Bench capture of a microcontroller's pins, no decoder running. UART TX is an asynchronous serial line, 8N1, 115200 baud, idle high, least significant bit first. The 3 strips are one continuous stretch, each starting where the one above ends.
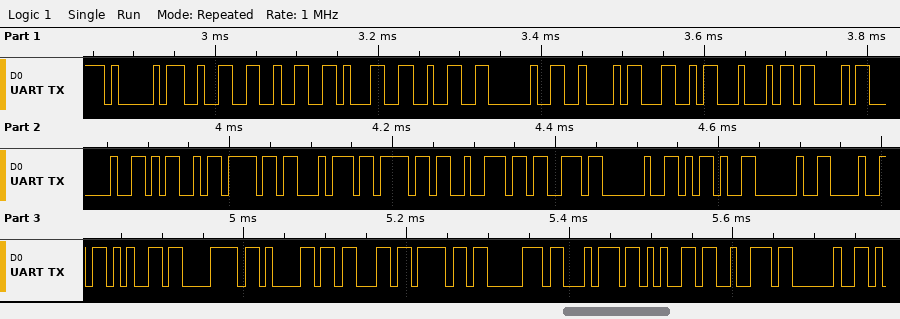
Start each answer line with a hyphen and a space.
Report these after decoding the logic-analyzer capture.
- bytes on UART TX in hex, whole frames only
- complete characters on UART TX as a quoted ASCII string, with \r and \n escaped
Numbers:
- 41 32 32 31 32 20 42 4C 44 43 20 4D 6F 74 6F 72 73 20 2D 20 48 65 78 61 63 6F 70 74 65 72 20
- "A2212 BLDC Motors - Hexacopter "
